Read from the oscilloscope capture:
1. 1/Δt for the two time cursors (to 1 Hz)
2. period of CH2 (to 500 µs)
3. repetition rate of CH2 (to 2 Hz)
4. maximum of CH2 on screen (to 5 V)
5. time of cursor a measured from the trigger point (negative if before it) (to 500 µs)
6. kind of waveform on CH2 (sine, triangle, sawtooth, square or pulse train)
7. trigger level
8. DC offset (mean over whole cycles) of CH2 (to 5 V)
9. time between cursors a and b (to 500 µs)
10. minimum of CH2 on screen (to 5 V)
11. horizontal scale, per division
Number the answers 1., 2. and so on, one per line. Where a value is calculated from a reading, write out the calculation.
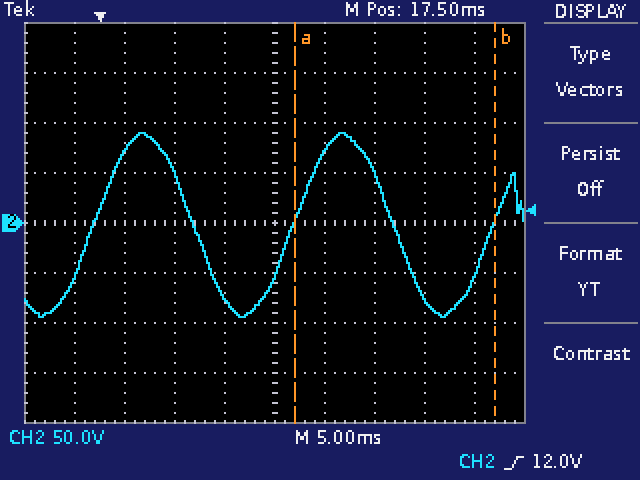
1. 1 / 20.0 ms ≈ 50 Hz
2. 20.0 ms
3. 1 / 20.0 ms ≈ 50 Hz
4. 90 V
5. +19.5 ms
6. sine
7. 12.0 V
8. (90 V + (-95 V)) / 2 ≈ 0 V
9. 20.0 ms
10. -95 V
11. 5 ms
